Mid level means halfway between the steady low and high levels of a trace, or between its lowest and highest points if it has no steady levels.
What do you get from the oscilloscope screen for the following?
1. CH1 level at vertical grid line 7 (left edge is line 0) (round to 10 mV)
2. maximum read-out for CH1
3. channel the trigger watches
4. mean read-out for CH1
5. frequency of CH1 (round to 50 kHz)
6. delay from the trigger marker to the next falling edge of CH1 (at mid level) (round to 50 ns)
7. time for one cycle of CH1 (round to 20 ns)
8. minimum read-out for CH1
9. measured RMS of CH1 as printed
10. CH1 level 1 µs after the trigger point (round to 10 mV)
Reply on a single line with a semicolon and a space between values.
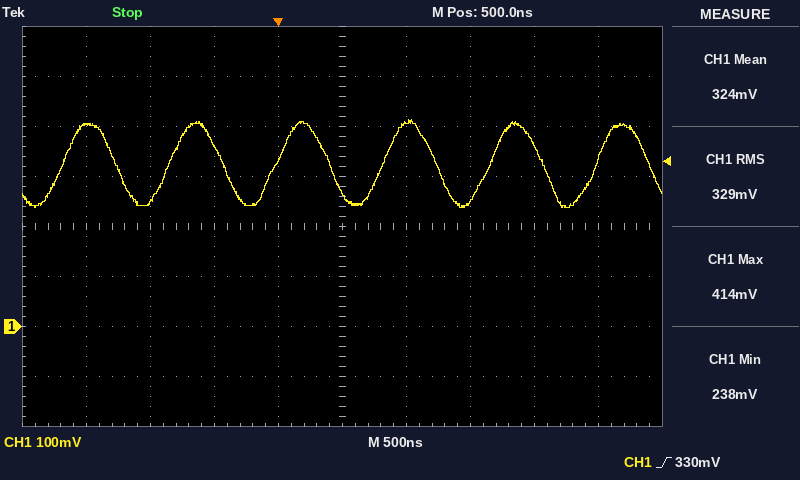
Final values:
250 mV; 414 mV; CH1; 324 mV; 1.20 MHz; 400 ns; 840 ns; 238 mV; 329 mV; 410 mV
